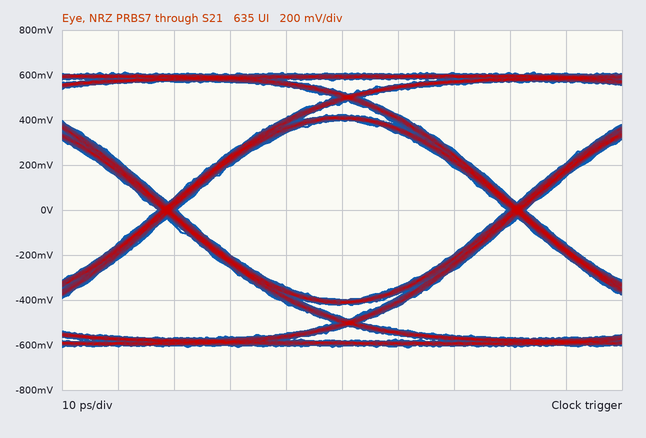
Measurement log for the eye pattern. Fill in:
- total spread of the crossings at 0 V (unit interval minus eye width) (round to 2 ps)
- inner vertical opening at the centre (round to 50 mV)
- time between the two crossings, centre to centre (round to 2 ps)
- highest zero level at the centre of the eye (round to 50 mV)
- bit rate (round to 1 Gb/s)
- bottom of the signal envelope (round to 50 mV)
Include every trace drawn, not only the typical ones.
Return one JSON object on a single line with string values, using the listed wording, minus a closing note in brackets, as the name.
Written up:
{"total spread of the crossings at 0 V (unit interval minus eye width)": "4 ps", "inner vertical opening at the centre": "800 mV", "time between the two crossings, centre to centre": "62 ps", "highest zero level at the centre of the eye": "-400 mV", "bit rate": "16 Gb/s", "bottom of the signal envelope": "-600 mV"}
